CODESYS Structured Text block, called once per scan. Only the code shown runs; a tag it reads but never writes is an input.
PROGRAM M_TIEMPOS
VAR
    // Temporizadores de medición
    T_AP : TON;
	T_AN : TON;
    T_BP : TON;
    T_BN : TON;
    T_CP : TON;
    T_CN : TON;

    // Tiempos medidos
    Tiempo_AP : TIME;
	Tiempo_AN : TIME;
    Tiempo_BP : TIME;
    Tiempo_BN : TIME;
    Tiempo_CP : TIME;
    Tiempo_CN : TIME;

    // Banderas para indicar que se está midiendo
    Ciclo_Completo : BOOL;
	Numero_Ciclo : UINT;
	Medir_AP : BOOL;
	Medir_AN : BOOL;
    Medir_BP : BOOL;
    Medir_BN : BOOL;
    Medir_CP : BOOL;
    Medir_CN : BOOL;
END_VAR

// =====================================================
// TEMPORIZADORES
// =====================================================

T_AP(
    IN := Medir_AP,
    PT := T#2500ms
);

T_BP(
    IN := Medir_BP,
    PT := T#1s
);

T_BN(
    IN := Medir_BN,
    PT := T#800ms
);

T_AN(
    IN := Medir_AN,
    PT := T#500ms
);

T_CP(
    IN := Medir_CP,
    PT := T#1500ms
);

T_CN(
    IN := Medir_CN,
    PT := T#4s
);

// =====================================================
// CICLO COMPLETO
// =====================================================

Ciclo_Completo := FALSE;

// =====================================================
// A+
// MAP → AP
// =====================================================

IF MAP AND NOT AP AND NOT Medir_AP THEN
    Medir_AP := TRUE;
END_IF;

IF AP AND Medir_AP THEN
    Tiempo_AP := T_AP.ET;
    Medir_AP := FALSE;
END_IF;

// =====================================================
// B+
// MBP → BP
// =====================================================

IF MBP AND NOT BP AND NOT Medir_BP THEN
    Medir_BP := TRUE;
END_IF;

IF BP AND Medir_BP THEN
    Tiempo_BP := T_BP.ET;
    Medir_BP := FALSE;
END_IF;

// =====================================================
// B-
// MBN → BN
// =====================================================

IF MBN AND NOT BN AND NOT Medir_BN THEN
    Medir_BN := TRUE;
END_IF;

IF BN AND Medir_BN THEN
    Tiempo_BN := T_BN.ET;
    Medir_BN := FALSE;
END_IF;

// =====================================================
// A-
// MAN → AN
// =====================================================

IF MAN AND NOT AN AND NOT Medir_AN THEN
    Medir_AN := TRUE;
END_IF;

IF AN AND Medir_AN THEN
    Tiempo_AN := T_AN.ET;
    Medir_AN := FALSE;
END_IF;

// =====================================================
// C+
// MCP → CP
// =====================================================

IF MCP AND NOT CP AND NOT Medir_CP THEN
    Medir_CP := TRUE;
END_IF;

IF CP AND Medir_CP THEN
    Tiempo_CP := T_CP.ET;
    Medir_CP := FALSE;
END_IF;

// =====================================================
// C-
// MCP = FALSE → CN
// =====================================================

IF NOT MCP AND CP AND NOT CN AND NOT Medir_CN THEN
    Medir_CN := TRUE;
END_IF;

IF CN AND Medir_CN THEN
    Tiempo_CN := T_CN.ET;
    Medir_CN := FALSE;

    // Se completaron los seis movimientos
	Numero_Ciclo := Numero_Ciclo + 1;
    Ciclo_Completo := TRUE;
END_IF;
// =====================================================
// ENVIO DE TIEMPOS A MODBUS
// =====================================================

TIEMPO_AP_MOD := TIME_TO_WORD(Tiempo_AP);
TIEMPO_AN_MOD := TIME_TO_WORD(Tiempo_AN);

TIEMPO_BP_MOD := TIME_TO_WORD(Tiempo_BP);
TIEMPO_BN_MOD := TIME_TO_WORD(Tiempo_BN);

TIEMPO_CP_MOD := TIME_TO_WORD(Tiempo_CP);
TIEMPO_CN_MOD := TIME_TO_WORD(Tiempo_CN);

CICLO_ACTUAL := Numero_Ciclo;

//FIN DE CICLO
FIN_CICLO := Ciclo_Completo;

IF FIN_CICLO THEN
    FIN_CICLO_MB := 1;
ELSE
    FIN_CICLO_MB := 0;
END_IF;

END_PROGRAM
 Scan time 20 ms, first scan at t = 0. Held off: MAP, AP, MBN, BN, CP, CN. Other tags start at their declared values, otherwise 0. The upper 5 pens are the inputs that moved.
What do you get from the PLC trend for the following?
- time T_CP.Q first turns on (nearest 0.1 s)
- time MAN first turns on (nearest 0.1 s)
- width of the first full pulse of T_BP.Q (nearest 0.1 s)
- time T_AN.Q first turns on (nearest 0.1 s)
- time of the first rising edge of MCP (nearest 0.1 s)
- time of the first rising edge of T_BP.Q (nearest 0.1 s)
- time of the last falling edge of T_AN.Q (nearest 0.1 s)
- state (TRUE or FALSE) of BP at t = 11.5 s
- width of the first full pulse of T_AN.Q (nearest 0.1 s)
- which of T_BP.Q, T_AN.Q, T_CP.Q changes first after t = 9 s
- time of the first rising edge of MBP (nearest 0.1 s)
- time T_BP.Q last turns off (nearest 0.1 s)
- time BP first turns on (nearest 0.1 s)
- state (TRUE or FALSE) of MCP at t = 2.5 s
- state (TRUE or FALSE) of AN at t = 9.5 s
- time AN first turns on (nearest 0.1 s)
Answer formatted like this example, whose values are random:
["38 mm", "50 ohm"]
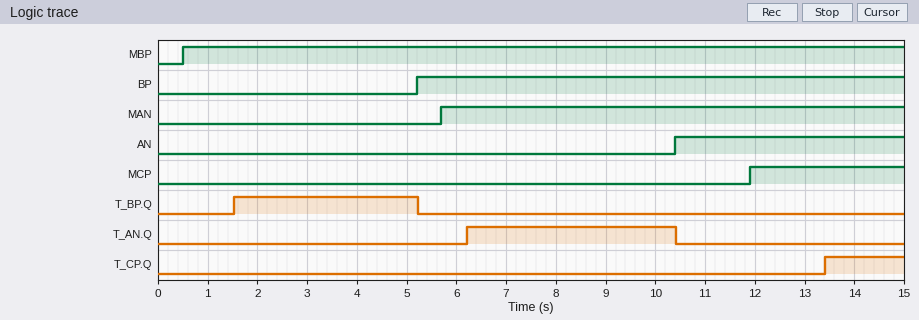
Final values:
["13.4 s", "5.7 s", "3.7 s", "6.2 s", "11.9 s", "1.5 s", "10.4 s", "TRUE", "4.2 s", "T_AN.Q", "0.5 s", "5.2 s", "5.2 s", "FALSE", "FALSE", "10.4 s"]
